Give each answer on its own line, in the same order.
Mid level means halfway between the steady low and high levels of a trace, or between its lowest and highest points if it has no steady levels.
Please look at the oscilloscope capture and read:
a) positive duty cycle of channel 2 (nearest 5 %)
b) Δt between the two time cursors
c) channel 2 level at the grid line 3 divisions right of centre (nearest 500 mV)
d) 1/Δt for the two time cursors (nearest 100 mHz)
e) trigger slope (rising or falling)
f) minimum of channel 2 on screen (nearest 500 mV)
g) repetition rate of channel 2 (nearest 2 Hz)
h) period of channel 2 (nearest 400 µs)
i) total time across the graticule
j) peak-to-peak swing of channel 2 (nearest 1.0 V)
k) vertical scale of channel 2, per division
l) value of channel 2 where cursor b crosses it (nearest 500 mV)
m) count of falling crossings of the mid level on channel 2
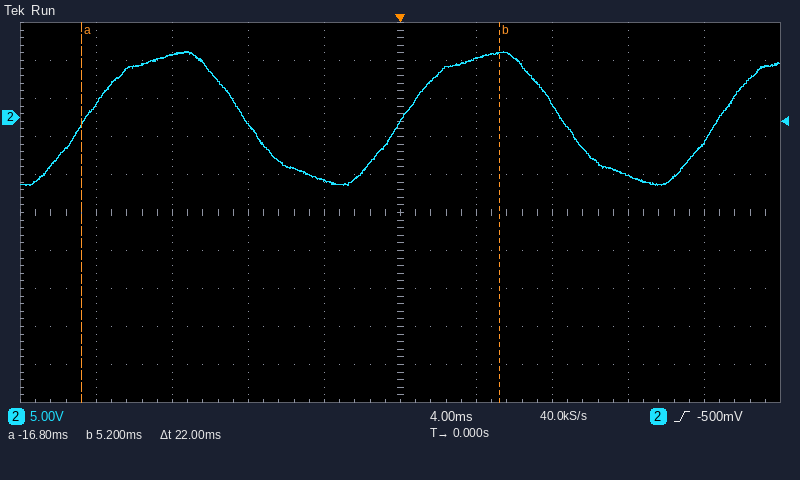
50 %
22 ms
-7.5 V
45.5 Hz
rising
-9.0 V
60 Hz
16.8 ms
40 ms
18.0 V
5 V
8.5 V
2
